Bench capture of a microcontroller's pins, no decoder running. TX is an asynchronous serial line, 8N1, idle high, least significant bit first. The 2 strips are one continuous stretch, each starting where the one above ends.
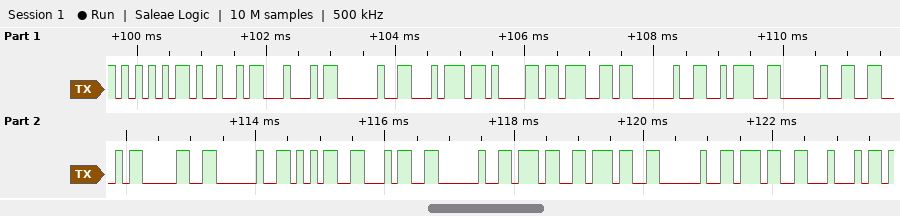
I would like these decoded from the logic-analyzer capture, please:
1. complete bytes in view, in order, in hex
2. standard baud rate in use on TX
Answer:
55 49 44 20 74 61 67 20 3A 20 46 30 20 35 34 20 37 37 20 37 44
9600 baud
